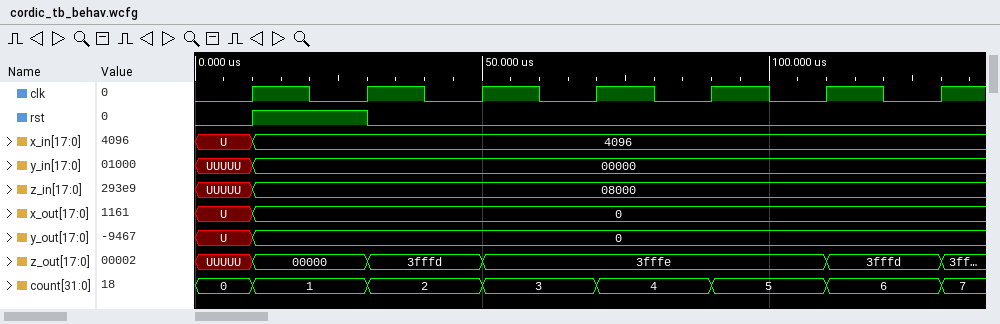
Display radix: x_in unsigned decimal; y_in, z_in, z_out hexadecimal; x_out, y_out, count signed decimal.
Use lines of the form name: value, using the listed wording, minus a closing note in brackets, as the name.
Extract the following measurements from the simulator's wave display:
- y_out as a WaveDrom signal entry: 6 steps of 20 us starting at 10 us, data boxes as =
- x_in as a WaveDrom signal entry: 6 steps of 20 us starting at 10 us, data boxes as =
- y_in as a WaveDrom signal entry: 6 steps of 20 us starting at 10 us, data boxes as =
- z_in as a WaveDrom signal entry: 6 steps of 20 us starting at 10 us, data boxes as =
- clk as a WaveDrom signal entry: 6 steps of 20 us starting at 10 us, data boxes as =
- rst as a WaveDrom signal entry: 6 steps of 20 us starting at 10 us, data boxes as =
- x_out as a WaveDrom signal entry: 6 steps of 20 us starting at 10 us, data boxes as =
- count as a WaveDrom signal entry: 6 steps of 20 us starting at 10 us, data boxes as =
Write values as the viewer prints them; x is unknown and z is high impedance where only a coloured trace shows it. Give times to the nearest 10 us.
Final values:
y_out as a WaveDrom signal entry: 6 steps of 20 us starting at 10 us, data boxes as =: {name: 'y_out', wave: '=.....', data: '0'}
x_in as a WaveDrom signal entry: 6 steps of 20 us starting at 10 us, data boxes as =: {name: 'x_in', wave: '=.....', data: '4096'}
y_in as a WaveDrom signal entry: 6 steps of 20 us starting at 10 us, data boxes as =: {name: 'y_in', wave: '=.....', data: '00000'}
z_in as a WaveDrom signal entry: 6 steps of 20 us starting at 10 us, data boxes as =: {name: 'z_in', wave: '=.....', data: '08000'}
clk as a WaveDrom signal entry: 6 steps of 20 us starting at 10 us, data boxes as =: {name: 'clk', wave: 'p.....'}
rst as a WaveDrom signal entry: 6 steps of 20 us starting at 10 us, data boxes as =: {name: 'rst', wave: '10....'}
x_out as a WaveDrom signal entry: 6 steps of 20 us starting at 10 us, data boxes as =: {name: 'x_out', wave: '=.....', data: '0'}
count as a WaveDrom signal entry: 6 steps of 20 us starting at 10 us, data boxes as =: {name: 'count', wave: '======', data: '1 2 3 4 5 6'}
